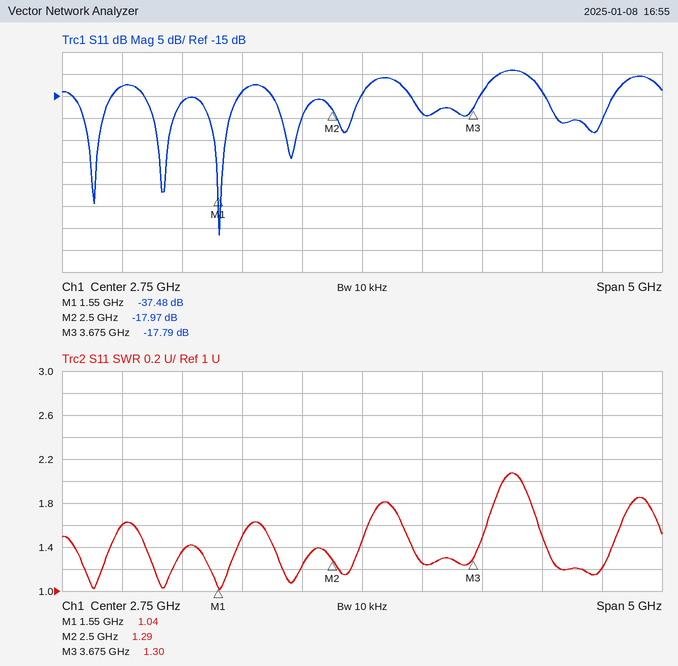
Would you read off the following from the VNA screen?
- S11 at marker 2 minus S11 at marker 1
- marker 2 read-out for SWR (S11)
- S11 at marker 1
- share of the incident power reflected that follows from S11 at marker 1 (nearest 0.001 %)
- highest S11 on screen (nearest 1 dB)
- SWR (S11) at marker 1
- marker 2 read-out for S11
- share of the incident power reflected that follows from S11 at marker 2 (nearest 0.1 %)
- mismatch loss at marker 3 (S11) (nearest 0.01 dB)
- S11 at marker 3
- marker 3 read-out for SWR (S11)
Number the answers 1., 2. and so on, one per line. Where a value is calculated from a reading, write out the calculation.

1. -17.97 − (-37.48) = 19.51 dB
2. 1.29
3. -37.48 dB
4. 10^(-37.48/10) ≈ 0.018 %
5. -9 dB
6. 1.04
7. -17.97 dB
8. 10^(-17.97/10) ≈ 1.6 %
9. −10 log10(1 − 10^(-17.79/10)) ≈ 0.07 dB
10. -17.79 dB
11. 1.30
